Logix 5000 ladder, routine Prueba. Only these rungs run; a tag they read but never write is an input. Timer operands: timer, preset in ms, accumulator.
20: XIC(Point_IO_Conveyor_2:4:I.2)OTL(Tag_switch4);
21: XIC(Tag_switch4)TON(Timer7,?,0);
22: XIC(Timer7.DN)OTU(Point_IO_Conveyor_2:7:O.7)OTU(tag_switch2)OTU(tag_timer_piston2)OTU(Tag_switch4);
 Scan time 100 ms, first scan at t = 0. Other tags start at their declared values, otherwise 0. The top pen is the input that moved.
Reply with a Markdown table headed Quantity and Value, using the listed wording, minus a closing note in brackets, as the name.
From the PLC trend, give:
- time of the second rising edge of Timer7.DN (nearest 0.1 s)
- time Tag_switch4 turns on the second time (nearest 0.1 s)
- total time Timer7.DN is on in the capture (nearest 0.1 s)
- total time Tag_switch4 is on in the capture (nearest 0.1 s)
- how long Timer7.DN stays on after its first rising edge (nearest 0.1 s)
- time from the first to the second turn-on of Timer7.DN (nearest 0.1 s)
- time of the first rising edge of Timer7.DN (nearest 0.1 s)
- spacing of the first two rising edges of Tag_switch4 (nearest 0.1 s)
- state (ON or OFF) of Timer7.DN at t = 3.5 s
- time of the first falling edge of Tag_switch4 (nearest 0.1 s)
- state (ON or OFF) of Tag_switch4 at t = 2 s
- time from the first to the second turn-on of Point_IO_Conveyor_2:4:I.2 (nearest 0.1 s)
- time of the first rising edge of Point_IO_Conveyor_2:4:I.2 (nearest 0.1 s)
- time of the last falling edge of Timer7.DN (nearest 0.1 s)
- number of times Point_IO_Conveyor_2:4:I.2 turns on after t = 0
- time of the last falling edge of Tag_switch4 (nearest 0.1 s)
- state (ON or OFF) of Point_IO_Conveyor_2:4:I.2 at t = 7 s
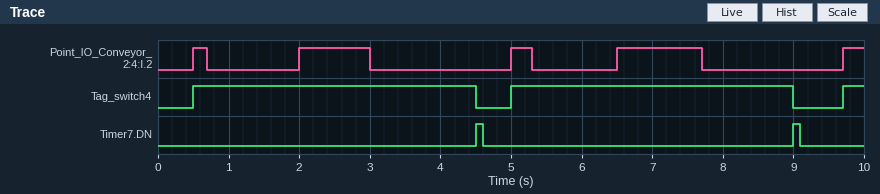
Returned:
| Quantity | Value |
|---|---|
| time of the second rising edge of Timer7.DN | 9.0 s |
| time Tag_switch4 turns on the second time | 5.0 s |
| total time Timer7.DN is on in the capture | 0.2 s |
| total time Tag_switch4 is on in the capture | 8.3 s |
| how long Timer7.DN stays on after its first rising edge | 0.1 s |
| time from the first to the second turn-on of Timer7.DN | 4.5 s |
| time of the first rising edge of Timer7.DN | 4.5 s |
| spacing of the first two rising edges of Tag_switch4 | 4.5 s |
| state (ON or OFF) of Timer7.DN at t = 3.5 s | OFF |
| time of the first falling edge of Tag_switch4 | 4.5 s |
| state (ON or OFF) of Tag_switch4 at t = 2 s | ON |
| time from the first to the second turn-on of Point_IO_Conveyor_2:4:I.2 | 1.5 s |
| time of the first rising edge of Point_IO_Conveyor_2:4:I.2 | 0.5 s |
| time of the last falling edge of Timer7.DN | 9.1 s |
| number of times Point_IO_Conveyor_2:4:I.2 turns on after t = 0 | 5 |
| time of the last falling edge of Tag_switch4 | 9.0 s |
| state (ON or OFF) of Point_IO_Conveyor_2:4:I.2 at t = 7 s | ON |
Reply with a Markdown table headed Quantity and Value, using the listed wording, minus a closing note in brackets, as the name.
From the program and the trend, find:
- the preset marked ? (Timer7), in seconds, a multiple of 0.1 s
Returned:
| Quantity | Value |
|---|---|
| the preset marked ? (Timer7), in seconds, a multiple of 0.1 s | 4.0 s |
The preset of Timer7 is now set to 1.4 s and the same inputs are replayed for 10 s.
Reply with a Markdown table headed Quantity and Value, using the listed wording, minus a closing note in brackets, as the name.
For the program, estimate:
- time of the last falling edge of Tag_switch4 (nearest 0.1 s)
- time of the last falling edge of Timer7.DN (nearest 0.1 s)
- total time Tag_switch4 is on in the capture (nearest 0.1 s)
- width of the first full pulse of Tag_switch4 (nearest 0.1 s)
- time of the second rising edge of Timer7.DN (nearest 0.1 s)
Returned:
| Quantity | Value |
|---|---|
| time of the last falling edge of Tag_switch4 | 6.4 s |
| time of the last falling edge of Timer7.DN | 7.7 s |
| total time Tag_switch4 is on in the capture | 3.1 s |
| width of the first full pulse of Tag_switch4 | 1.4 s |
| time of the second rising edge of Timer7.DN | 6.4 s |
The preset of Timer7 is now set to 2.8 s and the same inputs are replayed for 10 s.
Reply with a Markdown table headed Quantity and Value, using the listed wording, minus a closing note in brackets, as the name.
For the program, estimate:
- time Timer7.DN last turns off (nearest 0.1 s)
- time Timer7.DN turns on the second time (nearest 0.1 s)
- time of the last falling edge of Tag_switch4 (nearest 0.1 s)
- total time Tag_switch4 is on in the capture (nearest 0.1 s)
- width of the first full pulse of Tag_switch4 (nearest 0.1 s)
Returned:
| Quantity | Value |
|---|---|
| time Timer7.DN last turns off | 7.9 s |
| time Timer7.DN turns on the second time | 7.8 s |
| time of the last falling edge of Tag_switch4 | 7.8 s |
| total time Tag_switch4 is on in the capture | 5.9 s |
| width of the first full pulse of Tag_switch4 | 2.8 s |
